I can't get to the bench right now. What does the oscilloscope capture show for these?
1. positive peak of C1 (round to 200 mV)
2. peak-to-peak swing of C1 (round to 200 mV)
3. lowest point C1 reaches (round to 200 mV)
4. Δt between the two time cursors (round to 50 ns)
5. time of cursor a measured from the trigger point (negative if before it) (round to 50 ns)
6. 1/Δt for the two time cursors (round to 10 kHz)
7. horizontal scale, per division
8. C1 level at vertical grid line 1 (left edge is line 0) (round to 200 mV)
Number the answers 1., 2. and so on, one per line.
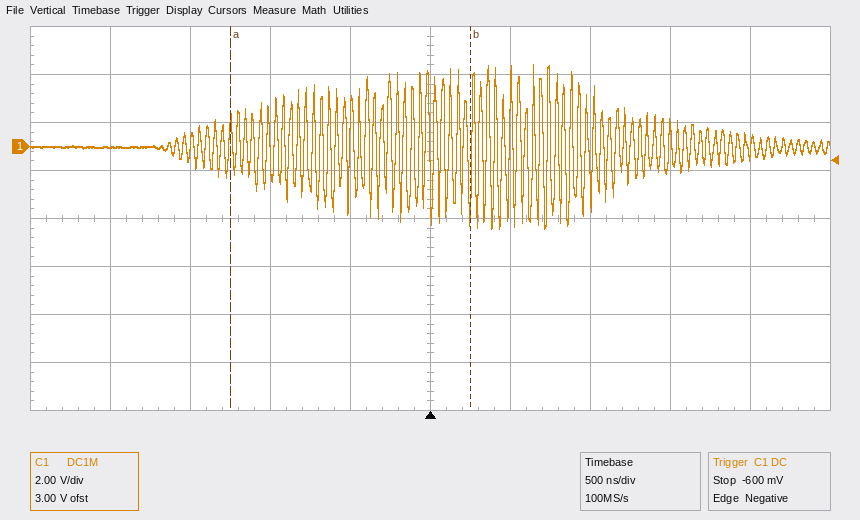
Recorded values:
1. 3.4 V
2. 6.8 V
3. -3.4 V
4. 1.50 µs
5. -1.25 µs
6. 670 kHz
7. 500 ns
8. 0.0 V
